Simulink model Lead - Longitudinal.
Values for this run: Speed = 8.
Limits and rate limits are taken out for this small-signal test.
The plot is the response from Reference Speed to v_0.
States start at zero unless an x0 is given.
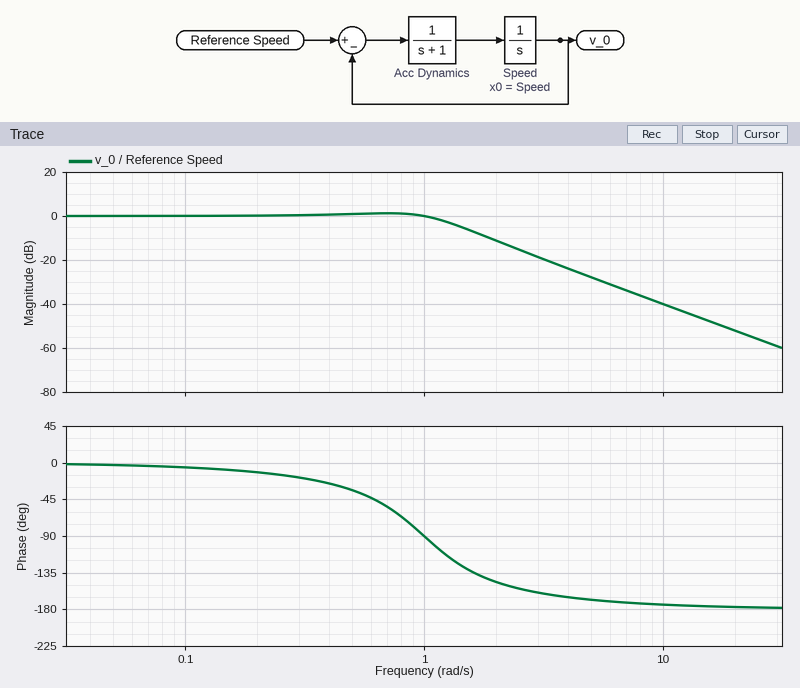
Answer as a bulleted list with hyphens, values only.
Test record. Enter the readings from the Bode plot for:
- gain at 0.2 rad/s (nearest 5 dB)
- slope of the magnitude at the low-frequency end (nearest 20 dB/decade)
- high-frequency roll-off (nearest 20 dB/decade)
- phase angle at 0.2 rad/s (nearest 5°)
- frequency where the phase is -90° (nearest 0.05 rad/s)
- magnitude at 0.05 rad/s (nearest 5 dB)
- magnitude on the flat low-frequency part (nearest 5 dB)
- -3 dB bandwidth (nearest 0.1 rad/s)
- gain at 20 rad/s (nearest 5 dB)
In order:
- 0 dB
- 0 dB/decade
- -40 dB/decade
- -10°
- 1.00 rad/s
- 0 dB
- 0 dB
- 1.3 rad/s
- -50 dB
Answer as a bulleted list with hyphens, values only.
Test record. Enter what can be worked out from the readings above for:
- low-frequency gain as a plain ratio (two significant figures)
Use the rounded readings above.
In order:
- 1.0
